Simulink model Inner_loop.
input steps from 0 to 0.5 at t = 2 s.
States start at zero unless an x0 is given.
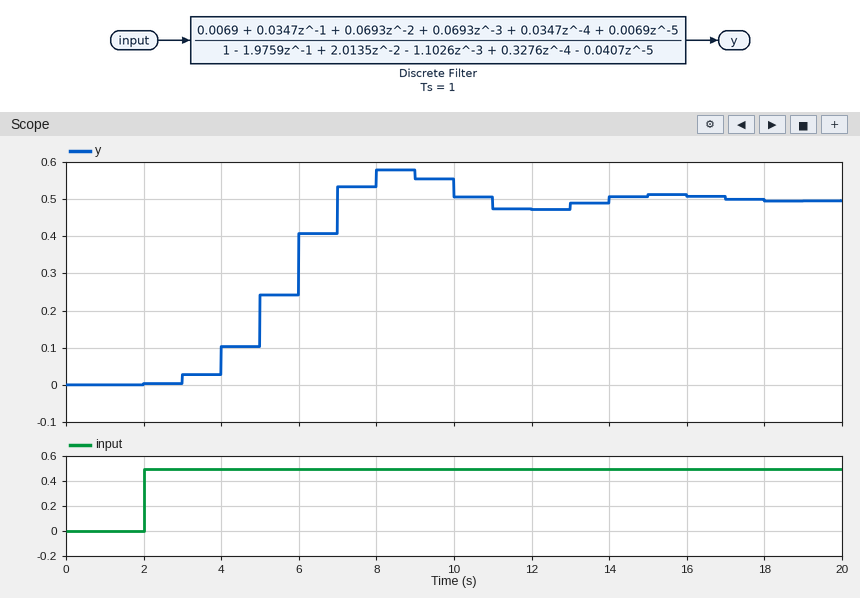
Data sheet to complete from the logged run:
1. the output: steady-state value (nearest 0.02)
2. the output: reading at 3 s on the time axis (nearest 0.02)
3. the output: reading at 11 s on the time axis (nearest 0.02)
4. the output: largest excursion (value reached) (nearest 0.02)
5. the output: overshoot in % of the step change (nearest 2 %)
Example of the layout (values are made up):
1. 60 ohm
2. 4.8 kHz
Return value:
1. 0.50
2. 0.02
3. 0.48
4. 0.58
5. 16 %
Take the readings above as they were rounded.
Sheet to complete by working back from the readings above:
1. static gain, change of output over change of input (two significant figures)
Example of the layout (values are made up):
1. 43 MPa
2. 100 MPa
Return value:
1. 1.0
